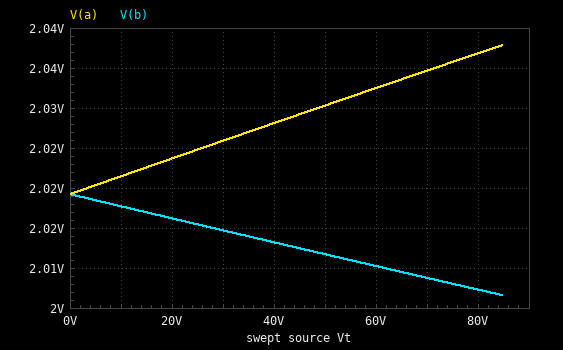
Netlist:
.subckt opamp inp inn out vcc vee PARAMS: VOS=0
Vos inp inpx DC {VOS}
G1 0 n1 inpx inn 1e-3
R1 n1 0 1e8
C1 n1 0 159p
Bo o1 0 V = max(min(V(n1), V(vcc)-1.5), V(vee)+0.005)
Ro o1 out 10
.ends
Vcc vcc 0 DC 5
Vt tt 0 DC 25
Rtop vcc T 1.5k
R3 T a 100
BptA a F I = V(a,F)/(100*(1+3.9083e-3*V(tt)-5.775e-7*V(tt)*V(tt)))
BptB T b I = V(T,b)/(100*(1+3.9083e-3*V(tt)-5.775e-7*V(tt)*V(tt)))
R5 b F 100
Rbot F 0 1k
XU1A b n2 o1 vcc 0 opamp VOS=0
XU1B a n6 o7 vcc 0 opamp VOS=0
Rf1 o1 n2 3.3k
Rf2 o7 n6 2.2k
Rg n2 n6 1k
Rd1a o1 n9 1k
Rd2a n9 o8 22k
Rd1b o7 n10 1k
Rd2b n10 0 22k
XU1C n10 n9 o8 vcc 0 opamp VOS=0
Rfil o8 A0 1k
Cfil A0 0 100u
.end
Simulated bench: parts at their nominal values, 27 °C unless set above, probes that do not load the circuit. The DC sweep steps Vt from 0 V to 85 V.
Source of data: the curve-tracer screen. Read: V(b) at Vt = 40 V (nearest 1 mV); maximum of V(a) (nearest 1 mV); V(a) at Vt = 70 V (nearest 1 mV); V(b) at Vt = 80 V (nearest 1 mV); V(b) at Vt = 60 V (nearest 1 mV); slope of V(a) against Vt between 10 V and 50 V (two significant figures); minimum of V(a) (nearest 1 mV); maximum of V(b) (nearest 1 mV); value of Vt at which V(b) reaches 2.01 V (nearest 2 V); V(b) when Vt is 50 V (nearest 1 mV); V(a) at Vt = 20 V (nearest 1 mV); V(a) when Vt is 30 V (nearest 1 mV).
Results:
2.013 V
2.038 V
2.035 V
2.007 V
2.010 V
0.00022 V/V
2.019 V
2.019 V
62 V
2.012 V
2.024 V
2.026 V
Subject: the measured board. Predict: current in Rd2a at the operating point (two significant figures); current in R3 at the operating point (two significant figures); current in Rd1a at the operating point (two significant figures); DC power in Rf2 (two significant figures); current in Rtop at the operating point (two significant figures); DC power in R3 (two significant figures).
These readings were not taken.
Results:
28 µA
960 µA
28 µA
190 nW
1.9 mA
92 µW
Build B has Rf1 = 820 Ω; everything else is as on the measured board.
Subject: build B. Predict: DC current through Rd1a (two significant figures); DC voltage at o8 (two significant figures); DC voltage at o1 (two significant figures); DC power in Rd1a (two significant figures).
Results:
51 µA
830 mV
2.0 V
2.6 µW
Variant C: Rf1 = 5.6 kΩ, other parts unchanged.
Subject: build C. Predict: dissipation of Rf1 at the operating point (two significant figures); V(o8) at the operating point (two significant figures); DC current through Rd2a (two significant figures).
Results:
490 nW
1.8 V
6.7 µA
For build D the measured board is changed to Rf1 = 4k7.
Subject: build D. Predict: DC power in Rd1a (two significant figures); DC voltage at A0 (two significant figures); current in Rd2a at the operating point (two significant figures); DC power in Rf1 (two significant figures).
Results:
230 nW
1.6 V
15 µA
410 nW
